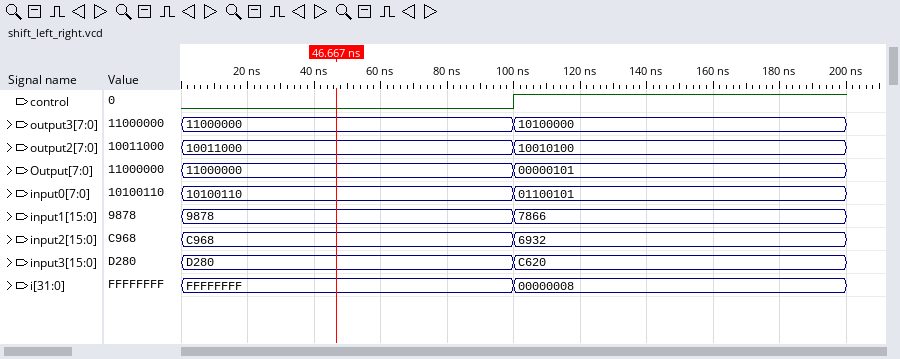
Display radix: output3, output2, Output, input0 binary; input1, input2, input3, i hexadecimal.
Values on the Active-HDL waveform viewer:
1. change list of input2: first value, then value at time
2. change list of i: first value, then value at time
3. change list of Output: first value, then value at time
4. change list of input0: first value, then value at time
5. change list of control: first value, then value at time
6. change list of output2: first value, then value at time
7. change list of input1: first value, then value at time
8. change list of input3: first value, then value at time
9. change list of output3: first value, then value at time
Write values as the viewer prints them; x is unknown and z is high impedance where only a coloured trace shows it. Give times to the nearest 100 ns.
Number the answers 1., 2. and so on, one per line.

1. C968, 6932 at 100 ns
2. FFFFFFFF, 00000008 at 100 ns
3. 11000000, 00000101 at 100 ns
4. 10100110, 01100101 at 100 ns
5. 0, 1 at 100 ns
6. 10011000, 10010100 at 100 ns
7. 9878, 7866 at 100 ns
8. D280, C620 at 100 ns
9. 11000000, 10100000 at 100 ns
